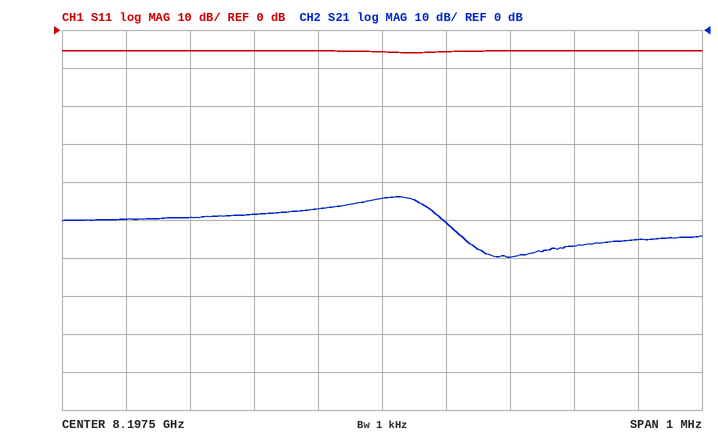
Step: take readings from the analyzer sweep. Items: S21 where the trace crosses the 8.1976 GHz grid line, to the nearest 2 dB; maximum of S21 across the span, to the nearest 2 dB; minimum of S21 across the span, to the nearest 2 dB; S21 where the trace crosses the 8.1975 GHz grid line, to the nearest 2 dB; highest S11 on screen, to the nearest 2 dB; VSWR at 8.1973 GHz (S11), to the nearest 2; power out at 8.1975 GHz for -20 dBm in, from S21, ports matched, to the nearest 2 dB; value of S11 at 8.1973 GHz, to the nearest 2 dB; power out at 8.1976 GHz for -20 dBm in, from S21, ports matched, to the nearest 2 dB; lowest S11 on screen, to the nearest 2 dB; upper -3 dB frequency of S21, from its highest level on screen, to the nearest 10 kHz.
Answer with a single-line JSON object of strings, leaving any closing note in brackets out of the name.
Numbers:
{"S21 where the trace crosses the 8.1976 GHz grid line, to the nearest 2 dB": "-50 dB", "maximum of S21 across the span, to the nearest 2 dB": "-44 dB", "minimum of S21 across the span, to the nearest 2 dB": "-60 dB", "S21 where the trace crosses the 8.1975 GHz grid line, to the nearest 2 dB": "-44 dB", "highest S11 on screen, to the nearest 2 dB": "-6 dB", "VSWR at 8.1973 GHz (S11), to the nearest 2": "4", "power out at 8.1975 GHz for -20 dBm in, from S21, ports matched, to the nearest 2 dB": "-64 dBm", "value of S11 at 8.1973 GHz, to the nearest 2 dB": "-6 dB", "power out at 8.1976 GHz for -20 dBm in, from S21, ports matched, to the nearest 2 dB": "-70 dBm", "lowest S11 on screen, to the nearest 2 dB": "-6 dB", "upper -3 dB frequency of S21, from its highest level on screen, to the nearest 10 kHz": "8.19757 GHz"}
